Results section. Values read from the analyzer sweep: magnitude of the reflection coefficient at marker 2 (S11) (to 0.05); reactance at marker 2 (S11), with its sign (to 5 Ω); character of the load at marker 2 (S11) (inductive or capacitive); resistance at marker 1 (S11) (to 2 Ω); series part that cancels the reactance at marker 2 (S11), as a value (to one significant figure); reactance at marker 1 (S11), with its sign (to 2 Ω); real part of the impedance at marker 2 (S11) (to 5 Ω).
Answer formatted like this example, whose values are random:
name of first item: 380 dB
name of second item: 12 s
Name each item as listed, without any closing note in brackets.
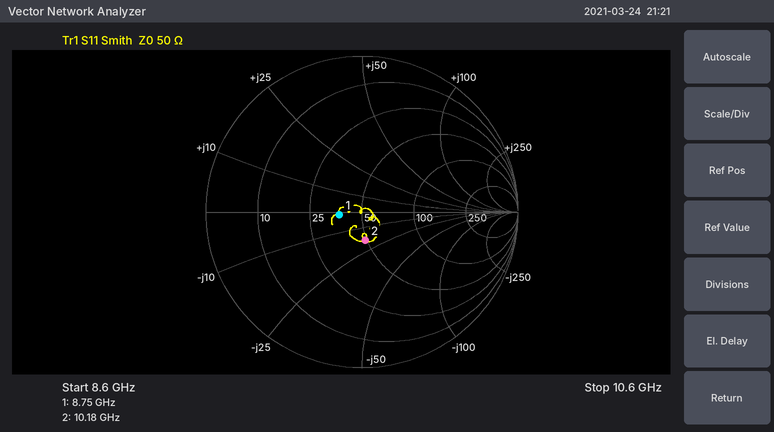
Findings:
magnitude of the reflection coefficient at marker 2 (S11): 0.20
reactance at marker 2 (S11), with its sign: -20 Ω
character of the load at marker 2 (S11): capacitive
resistance at marker 1 (S11): 38 Ω
series part that cancels the reactance at marker 2 (S11), as a value: 300 pH
reactance at marker 1 (S11), with its sign: -2 Ω
real part of the impedance at marker 2 (S11): 50 Ω
